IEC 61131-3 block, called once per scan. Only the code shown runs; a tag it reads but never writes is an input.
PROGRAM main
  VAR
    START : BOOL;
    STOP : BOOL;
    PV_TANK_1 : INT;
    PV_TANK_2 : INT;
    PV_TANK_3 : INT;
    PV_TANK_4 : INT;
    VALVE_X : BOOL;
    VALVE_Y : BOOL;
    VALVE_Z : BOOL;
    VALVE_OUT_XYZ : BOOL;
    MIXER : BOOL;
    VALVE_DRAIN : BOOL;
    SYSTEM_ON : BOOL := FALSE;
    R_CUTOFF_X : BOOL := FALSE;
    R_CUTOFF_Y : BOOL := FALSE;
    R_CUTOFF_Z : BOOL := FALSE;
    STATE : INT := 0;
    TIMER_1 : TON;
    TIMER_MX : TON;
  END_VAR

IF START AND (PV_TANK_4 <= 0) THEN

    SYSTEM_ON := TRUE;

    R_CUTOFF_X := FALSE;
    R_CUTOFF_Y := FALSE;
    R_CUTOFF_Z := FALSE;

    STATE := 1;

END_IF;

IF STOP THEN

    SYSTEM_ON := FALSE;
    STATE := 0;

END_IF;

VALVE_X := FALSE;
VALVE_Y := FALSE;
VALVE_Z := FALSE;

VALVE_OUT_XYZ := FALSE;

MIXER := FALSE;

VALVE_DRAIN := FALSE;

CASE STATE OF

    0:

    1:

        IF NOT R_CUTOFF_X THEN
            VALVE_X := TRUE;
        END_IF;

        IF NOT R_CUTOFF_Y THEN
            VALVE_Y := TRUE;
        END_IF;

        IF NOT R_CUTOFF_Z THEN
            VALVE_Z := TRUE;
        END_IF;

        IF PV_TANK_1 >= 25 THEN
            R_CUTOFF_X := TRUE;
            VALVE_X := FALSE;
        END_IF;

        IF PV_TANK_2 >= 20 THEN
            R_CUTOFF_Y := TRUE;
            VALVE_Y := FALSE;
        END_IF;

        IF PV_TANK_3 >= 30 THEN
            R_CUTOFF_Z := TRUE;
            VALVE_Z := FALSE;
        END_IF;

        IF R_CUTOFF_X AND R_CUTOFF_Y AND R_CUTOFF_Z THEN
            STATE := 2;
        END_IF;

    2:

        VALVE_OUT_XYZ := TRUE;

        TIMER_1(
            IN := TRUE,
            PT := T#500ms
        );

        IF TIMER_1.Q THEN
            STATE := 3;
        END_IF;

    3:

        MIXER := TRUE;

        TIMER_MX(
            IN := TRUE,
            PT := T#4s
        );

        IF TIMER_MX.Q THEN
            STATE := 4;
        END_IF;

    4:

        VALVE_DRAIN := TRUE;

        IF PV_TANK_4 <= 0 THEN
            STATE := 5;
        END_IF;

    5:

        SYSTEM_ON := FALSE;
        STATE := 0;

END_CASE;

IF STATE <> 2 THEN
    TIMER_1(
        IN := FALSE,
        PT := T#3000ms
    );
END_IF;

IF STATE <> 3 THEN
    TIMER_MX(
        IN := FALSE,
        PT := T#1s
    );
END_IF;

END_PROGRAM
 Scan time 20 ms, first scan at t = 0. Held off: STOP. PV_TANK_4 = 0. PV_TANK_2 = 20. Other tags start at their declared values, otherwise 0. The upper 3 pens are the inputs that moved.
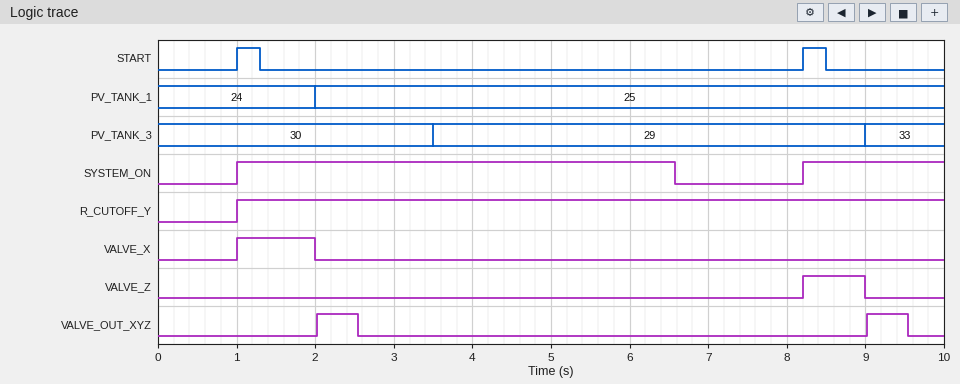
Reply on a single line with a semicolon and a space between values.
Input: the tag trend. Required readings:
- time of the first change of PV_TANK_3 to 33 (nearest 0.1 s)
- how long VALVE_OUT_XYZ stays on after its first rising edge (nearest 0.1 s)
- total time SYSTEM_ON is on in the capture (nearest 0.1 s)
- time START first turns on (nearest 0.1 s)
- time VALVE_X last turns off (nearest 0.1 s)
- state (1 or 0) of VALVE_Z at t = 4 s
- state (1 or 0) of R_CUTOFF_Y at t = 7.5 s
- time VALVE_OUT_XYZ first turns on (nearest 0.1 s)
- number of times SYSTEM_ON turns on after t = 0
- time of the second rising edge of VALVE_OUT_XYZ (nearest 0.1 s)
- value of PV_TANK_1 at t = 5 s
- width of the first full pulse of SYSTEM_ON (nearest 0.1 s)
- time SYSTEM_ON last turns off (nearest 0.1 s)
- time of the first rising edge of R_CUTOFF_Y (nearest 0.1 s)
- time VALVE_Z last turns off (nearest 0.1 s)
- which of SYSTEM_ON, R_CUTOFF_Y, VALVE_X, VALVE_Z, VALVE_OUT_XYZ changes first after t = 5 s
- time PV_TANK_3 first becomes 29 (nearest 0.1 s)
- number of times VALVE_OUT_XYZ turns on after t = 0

9.0 s; 0.5 s; 7.4 s; 1.0 s; 2.0 s; 0; 1; 2.0 s; 2; 9.0 s; 25; 5.6 s; 6.6 s; 1.0 s; 9.0 s; SYSTEM_ON; 3.5 s; 2
